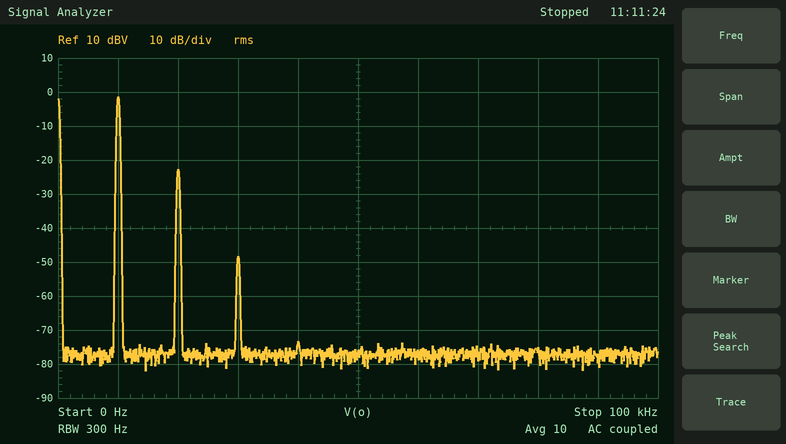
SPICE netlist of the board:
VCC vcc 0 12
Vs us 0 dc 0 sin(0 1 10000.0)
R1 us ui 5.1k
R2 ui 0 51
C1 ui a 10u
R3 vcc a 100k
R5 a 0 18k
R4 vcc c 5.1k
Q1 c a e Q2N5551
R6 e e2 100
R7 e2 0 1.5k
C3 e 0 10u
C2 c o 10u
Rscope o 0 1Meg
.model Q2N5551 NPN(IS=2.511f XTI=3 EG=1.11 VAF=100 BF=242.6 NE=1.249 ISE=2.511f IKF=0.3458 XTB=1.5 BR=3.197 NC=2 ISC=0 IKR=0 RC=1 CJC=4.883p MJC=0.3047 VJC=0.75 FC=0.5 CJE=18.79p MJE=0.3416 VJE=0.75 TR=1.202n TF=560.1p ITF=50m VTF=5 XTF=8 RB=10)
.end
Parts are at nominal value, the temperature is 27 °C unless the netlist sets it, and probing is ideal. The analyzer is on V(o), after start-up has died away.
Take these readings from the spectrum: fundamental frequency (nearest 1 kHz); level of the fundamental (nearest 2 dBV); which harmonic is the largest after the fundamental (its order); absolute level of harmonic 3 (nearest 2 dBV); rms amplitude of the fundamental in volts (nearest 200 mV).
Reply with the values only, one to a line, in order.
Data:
10 kHz
-2 dBV
2
-48 dBV
800 mV
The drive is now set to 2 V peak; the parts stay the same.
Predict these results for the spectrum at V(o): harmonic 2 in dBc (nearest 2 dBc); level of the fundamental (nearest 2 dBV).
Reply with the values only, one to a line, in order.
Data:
-16 dBc
4 dBV
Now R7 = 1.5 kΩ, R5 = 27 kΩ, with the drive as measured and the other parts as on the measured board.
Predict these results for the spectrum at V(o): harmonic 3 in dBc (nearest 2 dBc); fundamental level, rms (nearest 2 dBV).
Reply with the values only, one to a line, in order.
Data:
-48 dBc
2 dBV
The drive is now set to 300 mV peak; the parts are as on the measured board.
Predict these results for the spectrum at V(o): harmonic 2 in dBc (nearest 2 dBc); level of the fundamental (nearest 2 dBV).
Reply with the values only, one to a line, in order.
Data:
-32 dBc
-12 dBV
